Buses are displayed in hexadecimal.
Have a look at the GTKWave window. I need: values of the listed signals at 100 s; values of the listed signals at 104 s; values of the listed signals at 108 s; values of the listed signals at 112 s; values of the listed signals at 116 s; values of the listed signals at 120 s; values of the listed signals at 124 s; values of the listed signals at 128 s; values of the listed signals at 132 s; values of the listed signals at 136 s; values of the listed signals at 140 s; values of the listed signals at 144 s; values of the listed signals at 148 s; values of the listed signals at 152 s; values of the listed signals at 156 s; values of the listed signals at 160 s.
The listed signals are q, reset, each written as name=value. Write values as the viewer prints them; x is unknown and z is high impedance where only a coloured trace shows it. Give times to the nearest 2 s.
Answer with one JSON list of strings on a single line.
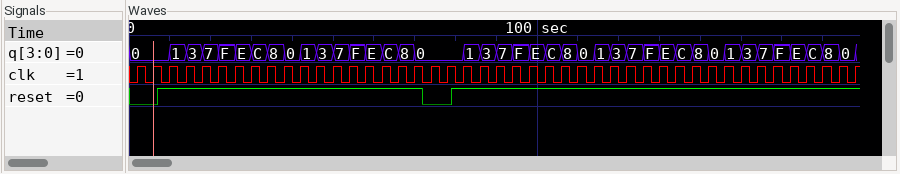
["q=E, reset=1", "q=C, reset=1", "q=8, reset=1", "q=0, reset=1", "q=1, reset=1", "q=3, reset=1", "q=7, reset=1", "q=F, reset=1", "q=E, reset=1", "q=C, reset=1", "q=8, reset=1", "q=0, reset=1", "q=1, reset=1", "q=3, reset=1", "q=7, reset=1", "q=F, reset=1"]
